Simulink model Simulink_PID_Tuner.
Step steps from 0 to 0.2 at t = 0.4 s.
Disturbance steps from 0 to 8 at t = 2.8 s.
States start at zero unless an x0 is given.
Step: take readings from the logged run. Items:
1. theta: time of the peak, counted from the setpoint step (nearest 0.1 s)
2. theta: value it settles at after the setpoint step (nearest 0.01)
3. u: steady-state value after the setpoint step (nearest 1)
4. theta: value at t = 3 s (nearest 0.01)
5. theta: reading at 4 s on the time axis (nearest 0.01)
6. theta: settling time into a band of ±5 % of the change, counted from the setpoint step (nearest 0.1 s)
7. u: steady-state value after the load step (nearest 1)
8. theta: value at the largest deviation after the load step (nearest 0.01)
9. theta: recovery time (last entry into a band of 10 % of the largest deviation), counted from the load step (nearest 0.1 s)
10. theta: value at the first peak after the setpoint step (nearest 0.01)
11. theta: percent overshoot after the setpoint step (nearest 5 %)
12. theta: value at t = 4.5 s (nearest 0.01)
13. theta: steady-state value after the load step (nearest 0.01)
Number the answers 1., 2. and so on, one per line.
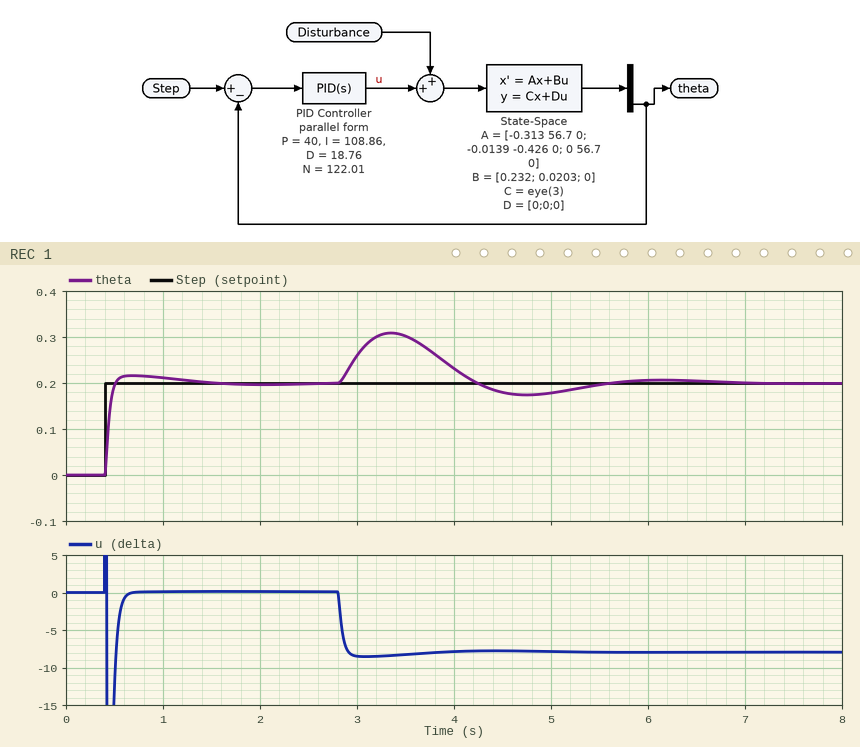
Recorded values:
1. 0.3 s
2. 0.20
3. 0
4. 0.26
5. 0.23
6. 0.7 s
7. -8
8. 0.31
9. 2.5 s
10. 0.22
11. 10 %
12. 0.18
13. 0.20
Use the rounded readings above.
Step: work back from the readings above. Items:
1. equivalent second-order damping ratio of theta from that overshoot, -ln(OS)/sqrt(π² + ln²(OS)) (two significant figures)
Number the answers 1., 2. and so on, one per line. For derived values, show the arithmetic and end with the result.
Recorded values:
1. ln(0.1) = -2.303; 2.303 / sqrt(9.870 + 5.302) = 0.59
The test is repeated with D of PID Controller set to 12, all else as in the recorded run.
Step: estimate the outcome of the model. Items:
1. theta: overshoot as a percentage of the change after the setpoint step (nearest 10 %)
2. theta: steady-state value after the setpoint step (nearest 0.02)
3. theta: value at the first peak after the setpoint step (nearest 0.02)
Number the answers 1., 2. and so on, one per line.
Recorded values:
1. 20 %
2. 0.20
3. 0.24
